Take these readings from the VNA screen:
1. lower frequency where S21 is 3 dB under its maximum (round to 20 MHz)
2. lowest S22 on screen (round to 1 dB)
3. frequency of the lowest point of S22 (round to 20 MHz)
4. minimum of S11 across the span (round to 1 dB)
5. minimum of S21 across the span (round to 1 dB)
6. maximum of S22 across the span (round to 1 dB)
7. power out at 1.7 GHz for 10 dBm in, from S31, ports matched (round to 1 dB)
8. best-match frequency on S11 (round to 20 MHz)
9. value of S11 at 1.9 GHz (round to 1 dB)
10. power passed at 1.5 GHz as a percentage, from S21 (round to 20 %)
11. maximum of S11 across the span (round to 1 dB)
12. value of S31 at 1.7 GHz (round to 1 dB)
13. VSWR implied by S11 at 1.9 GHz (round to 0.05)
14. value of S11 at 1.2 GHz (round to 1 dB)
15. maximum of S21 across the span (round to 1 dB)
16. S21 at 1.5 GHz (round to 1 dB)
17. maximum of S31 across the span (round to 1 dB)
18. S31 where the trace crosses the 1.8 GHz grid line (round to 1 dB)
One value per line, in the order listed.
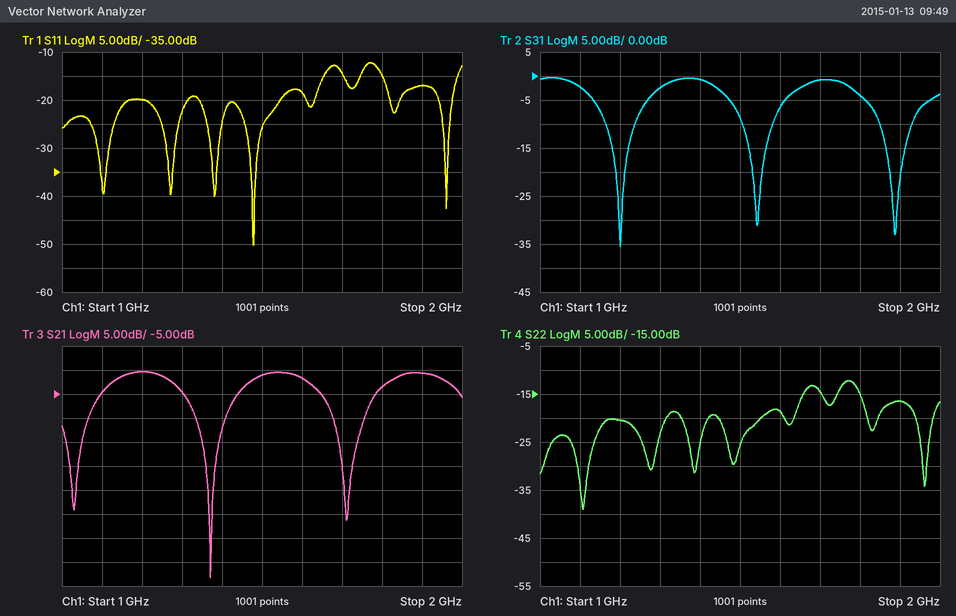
1.12 GHz
-39 dB
1.10 GHz
-50 dB
-43 dB
-12 dB
9 dBm
1.48 GHz
-17 dB
80 %
-12 dB
-1 dB
1.35
-20 dB
0 dB
-1 dB
0 dB
-4 dB
